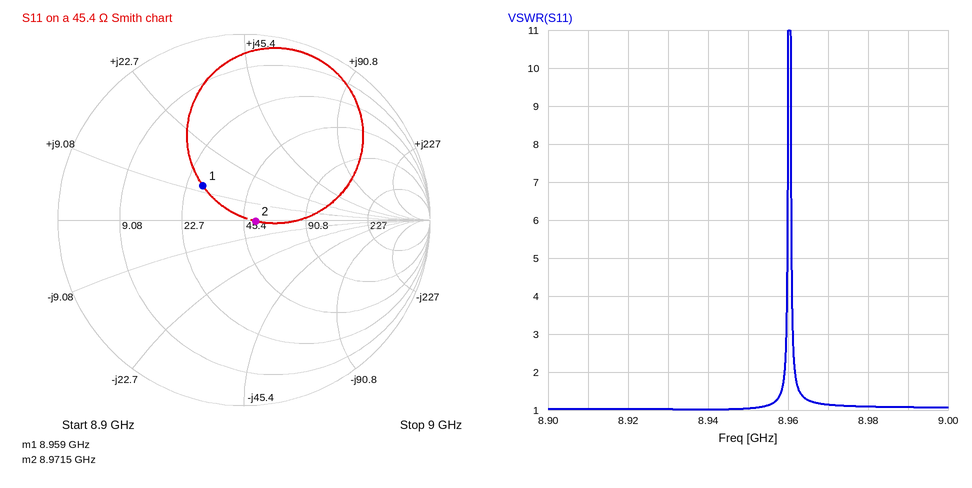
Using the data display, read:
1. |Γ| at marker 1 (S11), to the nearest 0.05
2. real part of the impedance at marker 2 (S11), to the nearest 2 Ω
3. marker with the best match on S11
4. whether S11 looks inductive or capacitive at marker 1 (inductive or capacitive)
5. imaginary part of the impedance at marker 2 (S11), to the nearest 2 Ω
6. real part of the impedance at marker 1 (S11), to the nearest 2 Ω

0.30
52 Ω
marker 2
inductive
0 Ω
28 Ω
